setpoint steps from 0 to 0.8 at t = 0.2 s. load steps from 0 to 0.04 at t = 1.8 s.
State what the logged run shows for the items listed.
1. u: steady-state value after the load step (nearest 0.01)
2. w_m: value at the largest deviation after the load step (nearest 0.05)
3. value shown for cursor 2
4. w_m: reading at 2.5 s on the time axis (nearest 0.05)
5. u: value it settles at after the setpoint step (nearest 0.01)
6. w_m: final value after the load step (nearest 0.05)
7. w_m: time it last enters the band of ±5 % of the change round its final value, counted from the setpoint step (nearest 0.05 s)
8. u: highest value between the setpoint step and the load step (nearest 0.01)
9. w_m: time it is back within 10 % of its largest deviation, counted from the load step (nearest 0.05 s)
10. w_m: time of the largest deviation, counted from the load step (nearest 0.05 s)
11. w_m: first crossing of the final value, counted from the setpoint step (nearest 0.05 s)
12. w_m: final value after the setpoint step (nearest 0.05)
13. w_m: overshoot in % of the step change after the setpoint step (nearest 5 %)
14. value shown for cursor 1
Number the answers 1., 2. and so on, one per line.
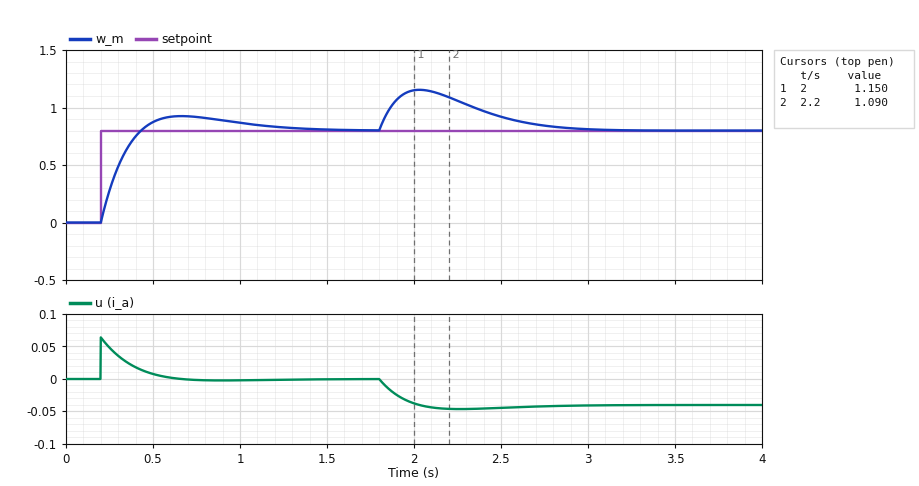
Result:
1. -0.04
2. 1.15
3. 1.090
4. 0.90
5. 0.00
6. 0.80
7. 0.95 s
8. 0.06
9. 1.00 s
10. 0.25 s
11. 0.25 s
12. 0.80
13. 15 %
14. 1.150
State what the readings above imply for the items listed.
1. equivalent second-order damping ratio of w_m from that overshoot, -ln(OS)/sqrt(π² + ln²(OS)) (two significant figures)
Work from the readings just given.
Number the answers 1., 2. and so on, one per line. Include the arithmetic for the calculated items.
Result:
1. ln(0.15) = -1.897; 1.897 / sqrt(9.870 + 3.599) = 0.52
